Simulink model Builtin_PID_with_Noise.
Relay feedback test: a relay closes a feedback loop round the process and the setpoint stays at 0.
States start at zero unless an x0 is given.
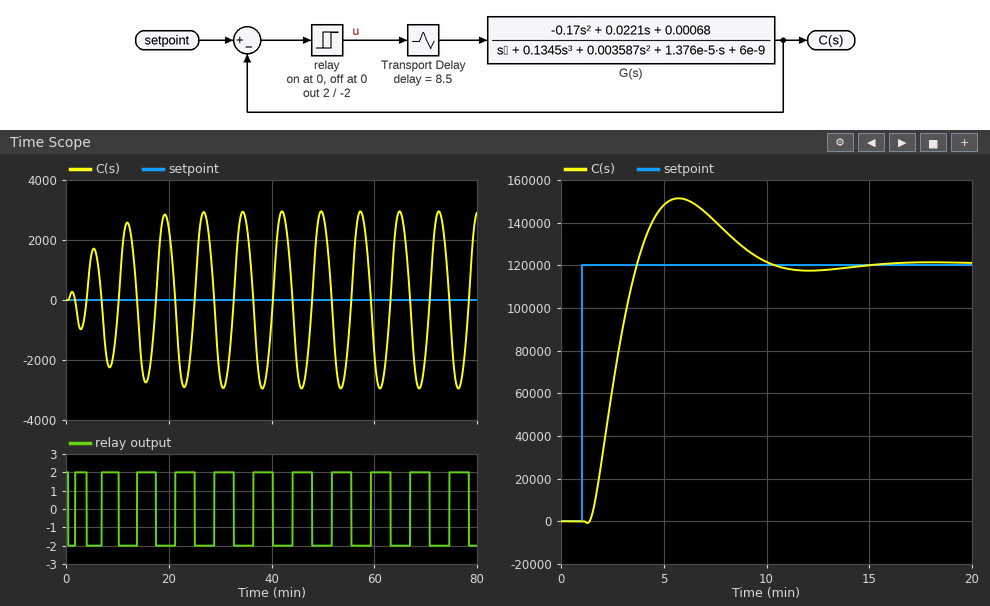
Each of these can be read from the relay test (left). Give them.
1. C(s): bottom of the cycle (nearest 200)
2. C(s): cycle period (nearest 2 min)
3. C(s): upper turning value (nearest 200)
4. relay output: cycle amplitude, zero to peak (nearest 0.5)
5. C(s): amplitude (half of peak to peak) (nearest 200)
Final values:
-3000
8 min
3000
2.0
3000
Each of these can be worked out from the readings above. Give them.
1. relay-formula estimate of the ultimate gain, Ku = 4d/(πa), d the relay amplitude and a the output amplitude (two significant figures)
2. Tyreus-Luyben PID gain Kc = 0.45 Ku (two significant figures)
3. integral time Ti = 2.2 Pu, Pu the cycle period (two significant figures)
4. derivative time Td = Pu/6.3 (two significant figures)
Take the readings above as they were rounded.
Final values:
0.00085
0.00038
18 min
1.3 min
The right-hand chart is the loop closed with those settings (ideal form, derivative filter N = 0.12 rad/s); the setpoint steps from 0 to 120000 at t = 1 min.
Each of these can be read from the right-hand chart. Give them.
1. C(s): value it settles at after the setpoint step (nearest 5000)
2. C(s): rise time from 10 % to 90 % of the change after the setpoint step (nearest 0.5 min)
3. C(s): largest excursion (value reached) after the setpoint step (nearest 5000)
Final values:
120000
1.5 min
150000
